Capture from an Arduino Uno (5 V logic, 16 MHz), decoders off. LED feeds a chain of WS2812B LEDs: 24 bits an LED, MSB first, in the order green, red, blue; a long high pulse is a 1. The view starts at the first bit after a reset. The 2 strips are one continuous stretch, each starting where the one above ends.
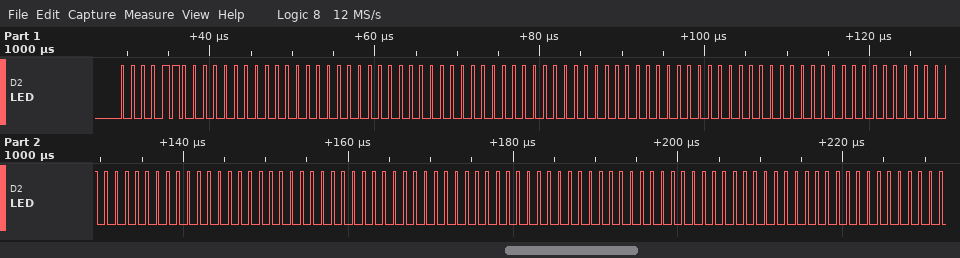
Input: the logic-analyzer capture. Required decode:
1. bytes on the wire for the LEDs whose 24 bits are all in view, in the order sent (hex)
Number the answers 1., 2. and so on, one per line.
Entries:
1. 0C 00 00 00 00 00 00 00 00 00 00 00 00 00 00 00 00 00
